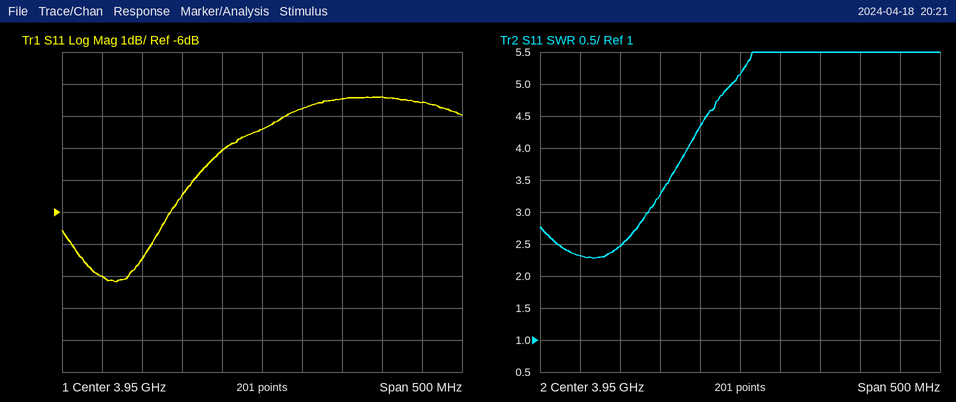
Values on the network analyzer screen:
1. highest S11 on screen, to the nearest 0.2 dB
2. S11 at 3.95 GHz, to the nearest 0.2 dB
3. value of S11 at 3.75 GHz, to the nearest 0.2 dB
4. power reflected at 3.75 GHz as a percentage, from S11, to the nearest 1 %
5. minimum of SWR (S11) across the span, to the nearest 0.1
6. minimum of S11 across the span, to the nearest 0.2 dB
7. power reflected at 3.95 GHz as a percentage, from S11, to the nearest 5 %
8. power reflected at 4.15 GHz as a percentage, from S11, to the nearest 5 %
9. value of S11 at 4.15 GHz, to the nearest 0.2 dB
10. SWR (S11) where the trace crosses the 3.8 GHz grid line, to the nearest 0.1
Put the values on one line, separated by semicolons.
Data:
-2.4 dB; -3.4 dB; -8.0 dB; 16 %; 2.3; -8.2 dB; 45 %; 55 %; -2.6 dB; 2.5
